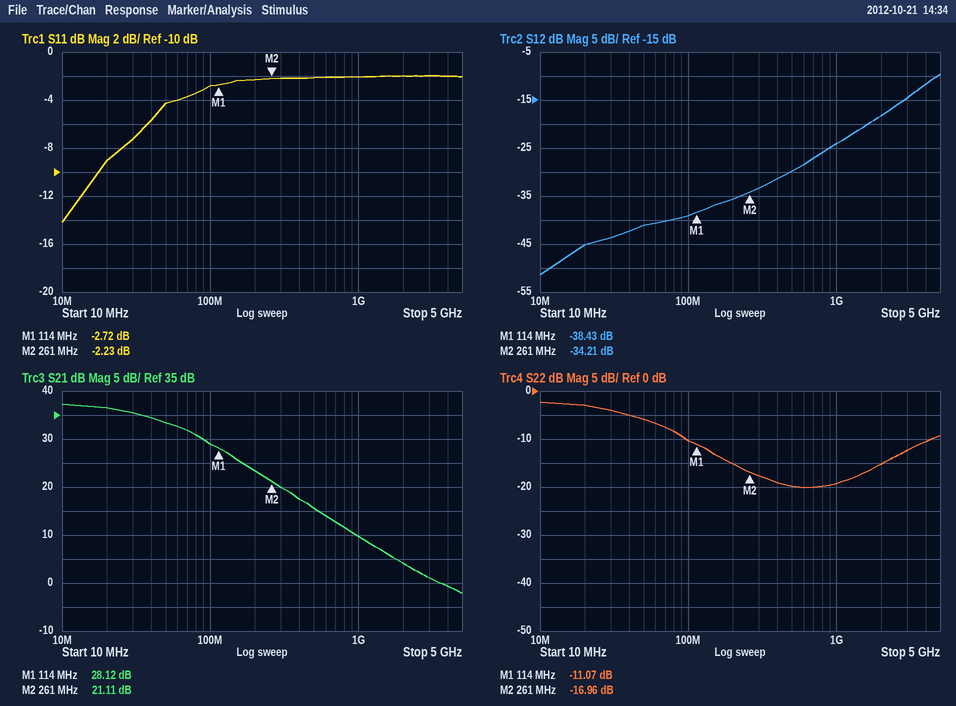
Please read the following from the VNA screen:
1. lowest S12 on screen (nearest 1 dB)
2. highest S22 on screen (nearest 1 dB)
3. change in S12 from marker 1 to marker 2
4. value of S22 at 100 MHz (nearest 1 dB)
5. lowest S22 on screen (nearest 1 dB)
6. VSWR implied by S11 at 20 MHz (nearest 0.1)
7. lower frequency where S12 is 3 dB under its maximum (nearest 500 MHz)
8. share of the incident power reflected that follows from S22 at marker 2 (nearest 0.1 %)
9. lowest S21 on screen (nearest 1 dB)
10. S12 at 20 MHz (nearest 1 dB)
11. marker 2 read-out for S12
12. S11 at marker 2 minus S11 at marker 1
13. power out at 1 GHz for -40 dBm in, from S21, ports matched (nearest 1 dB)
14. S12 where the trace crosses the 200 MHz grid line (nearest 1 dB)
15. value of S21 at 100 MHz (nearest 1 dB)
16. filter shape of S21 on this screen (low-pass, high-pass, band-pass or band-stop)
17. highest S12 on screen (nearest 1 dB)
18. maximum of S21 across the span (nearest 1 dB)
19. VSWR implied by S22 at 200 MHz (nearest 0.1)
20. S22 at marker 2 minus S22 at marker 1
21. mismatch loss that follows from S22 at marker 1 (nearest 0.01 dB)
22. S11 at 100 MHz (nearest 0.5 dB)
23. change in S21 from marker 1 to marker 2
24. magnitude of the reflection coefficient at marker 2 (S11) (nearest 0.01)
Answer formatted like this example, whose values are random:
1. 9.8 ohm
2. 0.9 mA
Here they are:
1. -51 dB
2. -2 dB
3. 4.22 dB
4. -10 dB
5. -20 dB
6. 2.1
7. 3.5 GHz
8. 2.0 %
9. -2 dB
10. -45 dB
11. -34.21 dB
12. 0.49 dB
13. -30 dBm
14. -36 dB
15. 29 dB
16. low-pass
17. -10 dB
18. 37 dB
19. 1.4
20. -5.89 dB
21. 0.35 dB
22. -3.0 dB
23. -7.01 dB
24. 0.77
